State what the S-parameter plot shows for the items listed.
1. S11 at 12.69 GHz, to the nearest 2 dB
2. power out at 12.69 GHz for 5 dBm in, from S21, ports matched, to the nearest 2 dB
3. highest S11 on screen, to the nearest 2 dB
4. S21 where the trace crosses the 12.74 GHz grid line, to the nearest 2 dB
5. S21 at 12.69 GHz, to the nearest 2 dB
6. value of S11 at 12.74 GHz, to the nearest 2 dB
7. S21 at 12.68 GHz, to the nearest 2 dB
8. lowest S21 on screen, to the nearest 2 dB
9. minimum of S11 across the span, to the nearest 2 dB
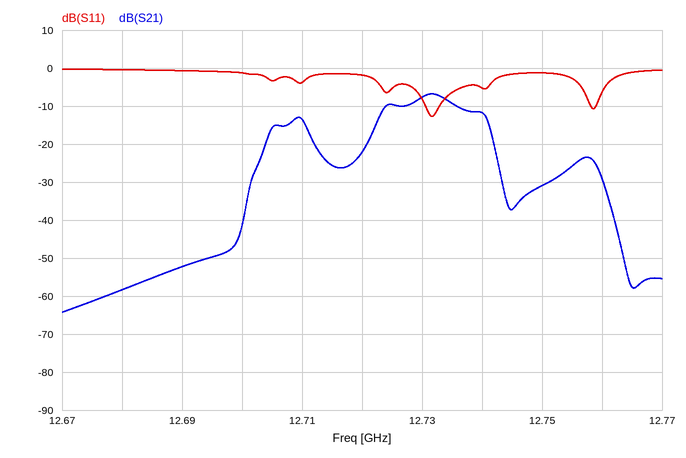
0 dB
-48 dBm
0 dB
-12 dB
-52 dB
-6 dB
-58 dB
-64 dB
-12 dB
